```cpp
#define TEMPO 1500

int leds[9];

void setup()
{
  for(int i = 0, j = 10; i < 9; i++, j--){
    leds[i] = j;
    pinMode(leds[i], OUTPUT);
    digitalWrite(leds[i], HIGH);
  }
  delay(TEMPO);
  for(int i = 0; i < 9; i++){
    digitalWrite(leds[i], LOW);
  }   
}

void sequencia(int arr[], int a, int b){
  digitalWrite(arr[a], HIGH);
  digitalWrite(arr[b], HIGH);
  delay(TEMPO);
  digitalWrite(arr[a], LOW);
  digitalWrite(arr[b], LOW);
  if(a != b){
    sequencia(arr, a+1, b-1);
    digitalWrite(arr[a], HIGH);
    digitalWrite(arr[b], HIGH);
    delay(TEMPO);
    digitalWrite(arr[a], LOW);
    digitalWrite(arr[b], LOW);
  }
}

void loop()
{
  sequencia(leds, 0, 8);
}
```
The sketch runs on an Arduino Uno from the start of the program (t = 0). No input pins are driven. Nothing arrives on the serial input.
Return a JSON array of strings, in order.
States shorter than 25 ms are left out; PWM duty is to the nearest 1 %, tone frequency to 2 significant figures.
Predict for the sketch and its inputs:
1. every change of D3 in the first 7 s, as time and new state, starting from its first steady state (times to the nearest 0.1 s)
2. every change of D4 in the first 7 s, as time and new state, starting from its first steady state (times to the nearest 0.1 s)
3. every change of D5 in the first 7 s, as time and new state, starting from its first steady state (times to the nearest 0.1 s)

["0 s high; 1.5 s low; 3 s high; 4.5 s low", "0 s high; 1.5 s low; 4.5 s high; 6 s low", "0 s high; 1.5 s low; 6 s high"]
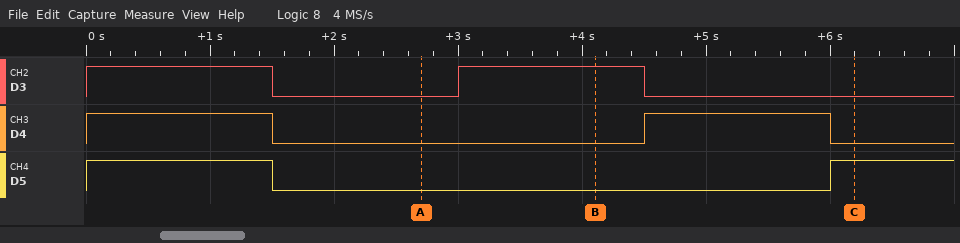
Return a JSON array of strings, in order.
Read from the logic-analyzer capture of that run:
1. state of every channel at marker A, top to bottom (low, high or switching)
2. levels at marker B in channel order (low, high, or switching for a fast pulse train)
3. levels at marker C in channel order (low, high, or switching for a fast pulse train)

["D3 low, D4 low, D5 low", "D3 high, D4 low, D5 low", "D3 low, D4 low, D5 high"]
